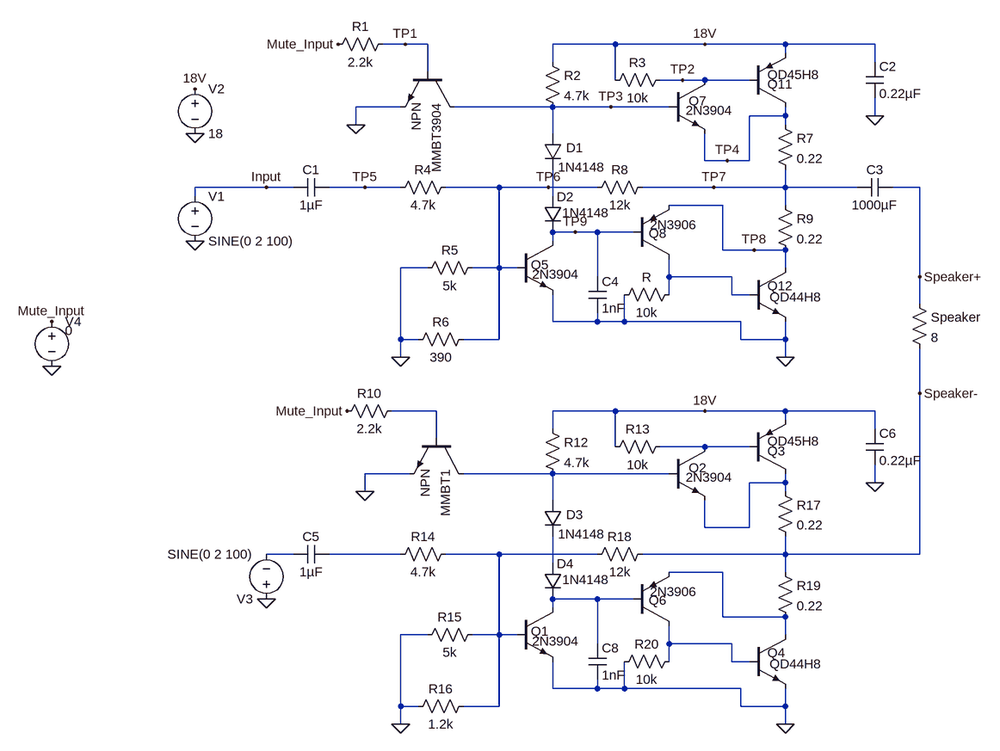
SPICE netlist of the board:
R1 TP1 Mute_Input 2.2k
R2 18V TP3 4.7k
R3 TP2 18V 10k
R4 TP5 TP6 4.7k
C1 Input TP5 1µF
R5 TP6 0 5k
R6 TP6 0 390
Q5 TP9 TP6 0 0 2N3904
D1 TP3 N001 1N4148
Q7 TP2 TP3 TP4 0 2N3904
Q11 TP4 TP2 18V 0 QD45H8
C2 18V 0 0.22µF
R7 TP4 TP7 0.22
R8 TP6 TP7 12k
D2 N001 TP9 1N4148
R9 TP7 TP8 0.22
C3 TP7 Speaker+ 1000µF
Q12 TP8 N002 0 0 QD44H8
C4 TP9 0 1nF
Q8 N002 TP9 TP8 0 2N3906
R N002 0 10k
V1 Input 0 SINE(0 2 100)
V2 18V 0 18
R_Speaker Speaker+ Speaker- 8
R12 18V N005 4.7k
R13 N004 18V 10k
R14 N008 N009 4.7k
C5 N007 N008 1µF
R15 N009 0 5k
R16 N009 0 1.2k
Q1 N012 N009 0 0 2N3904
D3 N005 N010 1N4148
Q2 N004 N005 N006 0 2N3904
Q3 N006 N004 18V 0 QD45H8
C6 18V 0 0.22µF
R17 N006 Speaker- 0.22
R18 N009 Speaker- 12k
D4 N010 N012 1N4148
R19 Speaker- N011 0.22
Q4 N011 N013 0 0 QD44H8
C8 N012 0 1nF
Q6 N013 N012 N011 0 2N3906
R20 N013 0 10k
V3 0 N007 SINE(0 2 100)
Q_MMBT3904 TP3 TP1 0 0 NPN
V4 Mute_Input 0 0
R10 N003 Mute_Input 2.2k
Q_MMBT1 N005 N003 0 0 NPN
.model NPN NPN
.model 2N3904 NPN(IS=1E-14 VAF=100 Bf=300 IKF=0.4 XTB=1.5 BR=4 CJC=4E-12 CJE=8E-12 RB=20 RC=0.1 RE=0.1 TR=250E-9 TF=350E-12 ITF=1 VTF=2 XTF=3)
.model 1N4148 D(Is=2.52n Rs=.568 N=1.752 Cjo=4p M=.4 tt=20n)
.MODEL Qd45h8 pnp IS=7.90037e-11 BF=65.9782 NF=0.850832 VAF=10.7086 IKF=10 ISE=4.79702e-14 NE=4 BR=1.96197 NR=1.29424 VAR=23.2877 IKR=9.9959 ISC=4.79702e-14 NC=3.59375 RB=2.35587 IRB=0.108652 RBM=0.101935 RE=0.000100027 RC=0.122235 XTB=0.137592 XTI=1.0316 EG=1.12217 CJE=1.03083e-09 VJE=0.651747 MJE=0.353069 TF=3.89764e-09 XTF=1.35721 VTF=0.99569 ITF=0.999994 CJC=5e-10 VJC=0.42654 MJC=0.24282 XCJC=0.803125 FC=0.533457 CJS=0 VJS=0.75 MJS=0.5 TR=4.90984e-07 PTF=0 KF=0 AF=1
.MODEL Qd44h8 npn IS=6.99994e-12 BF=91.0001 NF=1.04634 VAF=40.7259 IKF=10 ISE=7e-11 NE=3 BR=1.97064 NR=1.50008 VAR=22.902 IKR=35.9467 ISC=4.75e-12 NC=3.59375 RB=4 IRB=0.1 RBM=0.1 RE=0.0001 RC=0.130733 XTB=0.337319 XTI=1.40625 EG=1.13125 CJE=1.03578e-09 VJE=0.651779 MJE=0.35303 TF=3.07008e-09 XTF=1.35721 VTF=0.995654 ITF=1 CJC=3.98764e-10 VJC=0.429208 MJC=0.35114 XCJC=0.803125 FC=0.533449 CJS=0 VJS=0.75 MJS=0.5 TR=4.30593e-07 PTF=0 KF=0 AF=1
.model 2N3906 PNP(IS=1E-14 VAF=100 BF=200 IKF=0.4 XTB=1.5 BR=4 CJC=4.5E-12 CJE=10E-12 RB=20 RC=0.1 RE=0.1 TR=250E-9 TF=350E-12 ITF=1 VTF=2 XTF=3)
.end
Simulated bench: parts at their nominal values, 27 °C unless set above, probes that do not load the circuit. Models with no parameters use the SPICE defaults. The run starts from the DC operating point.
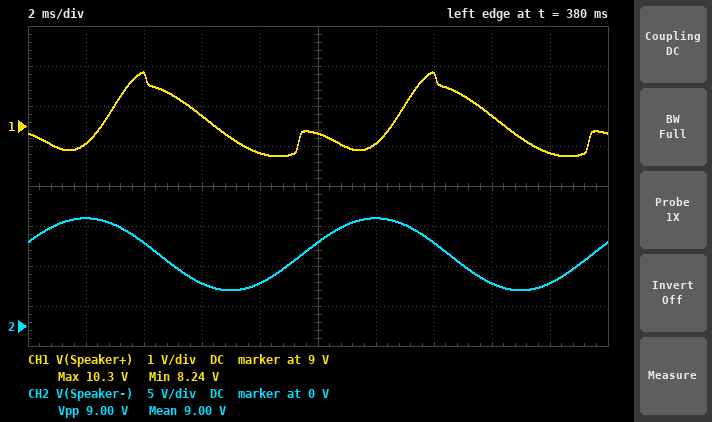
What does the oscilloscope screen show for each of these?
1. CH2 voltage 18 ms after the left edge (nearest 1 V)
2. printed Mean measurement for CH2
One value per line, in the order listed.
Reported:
5 V
9.00 V
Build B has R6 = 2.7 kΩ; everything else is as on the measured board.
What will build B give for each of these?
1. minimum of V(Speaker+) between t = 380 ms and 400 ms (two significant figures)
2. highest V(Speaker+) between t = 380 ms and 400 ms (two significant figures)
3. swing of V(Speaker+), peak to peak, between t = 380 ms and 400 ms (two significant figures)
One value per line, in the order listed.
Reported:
4.3 V
14 V
9.3 V
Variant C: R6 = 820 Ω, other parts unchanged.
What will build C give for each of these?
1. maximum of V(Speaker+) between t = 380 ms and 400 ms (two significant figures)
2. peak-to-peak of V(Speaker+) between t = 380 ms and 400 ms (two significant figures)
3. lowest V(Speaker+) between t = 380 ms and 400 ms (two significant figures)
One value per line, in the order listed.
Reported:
13 V
8.4 V
4.7 V
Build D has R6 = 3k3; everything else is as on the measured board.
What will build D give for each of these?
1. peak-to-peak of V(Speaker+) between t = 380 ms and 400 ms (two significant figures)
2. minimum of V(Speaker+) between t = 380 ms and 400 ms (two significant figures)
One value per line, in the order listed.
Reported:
9.1 V
4.4 V
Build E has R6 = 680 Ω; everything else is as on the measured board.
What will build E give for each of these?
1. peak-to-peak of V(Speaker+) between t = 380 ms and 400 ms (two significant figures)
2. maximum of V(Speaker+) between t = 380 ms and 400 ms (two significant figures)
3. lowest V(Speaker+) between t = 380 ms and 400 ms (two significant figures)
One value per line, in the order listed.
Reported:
7.6 V
13 V
5.0 V
